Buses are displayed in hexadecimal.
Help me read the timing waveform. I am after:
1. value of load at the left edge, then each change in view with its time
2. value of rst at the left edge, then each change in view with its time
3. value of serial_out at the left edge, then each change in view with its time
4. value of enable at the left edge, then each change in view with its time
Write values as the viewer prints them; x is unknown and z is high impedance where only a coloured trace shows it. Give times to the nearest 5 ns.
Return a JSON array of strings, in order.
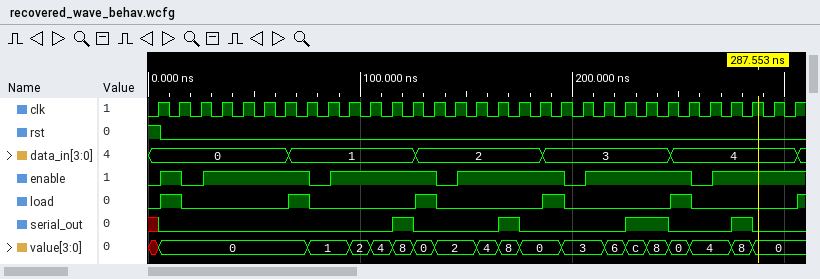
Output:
["0, 1 at 5 ns, 0 at 15 ns, 1 at 65 ns, 0 at 75 ns, 1 at 125 ns, 0 at 135 ns, 1 at 185 ns, 0 at 195 ns, 1 at 245 ns, 0 at 255 ns, 1 at 305 ns", "1, 0 at 5 ns", "x, 0 at 5 ns, 1 at 115 ns, 0 at 125 ns, 1 at 165 ns, 0 at 175 ns, 1 at 225 ns, 0 at 245 ns, 1 at 275 ns, 0 at 285 ns", "0, 1 at 5 ns, 0 at 15 ns, 1 at 25 ns, 0 at 75 ns, 1 at 85 ns, 0 at 135 ns, 1 at 145 ns, 0 at 195 ns, 1 at 205 ns, 0 at 255 ns, 1 at 265 ns"]
